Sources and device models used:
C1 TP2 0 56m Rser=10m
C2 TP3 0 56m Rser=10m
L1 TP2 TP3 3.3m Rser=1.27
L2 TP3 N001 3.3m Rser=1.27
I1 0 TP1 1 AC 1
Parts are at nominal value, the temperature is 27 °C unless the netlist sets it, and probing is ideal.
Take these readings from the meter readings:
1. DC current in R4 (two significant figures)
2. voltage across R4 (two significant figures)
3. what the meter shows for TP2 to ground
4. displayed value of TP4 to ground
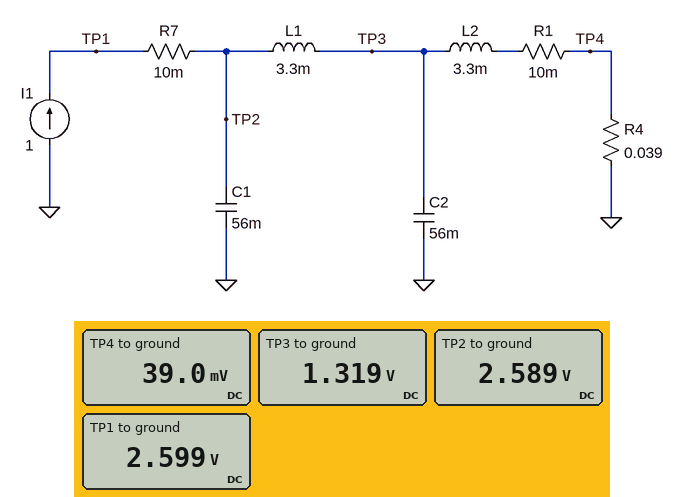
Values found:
1.0 A
39 mV
2.589 V
39.0 mV
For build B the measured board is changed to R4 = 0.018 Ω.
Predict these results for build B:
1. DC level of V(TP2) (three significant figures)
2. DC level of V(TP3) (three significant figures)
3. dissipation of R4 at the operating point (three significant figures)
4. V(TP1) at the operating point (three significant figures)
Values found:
2.57 V
1.30 V
18.0 mW
2.58 V
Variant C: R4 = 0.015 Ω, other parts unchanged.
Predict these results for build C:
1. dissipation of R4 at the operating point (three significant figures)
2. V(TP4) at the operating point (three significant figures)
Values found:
15.0 mW
15.0 mV
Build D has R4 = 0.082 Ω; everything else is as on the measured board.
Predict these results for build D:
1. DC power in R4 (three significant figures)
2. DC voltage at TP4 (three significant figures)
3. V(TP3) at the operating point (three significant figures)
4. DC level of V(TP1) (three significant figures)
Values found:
82.0 mW
82.0 mV
1.36 V
2.64 V
